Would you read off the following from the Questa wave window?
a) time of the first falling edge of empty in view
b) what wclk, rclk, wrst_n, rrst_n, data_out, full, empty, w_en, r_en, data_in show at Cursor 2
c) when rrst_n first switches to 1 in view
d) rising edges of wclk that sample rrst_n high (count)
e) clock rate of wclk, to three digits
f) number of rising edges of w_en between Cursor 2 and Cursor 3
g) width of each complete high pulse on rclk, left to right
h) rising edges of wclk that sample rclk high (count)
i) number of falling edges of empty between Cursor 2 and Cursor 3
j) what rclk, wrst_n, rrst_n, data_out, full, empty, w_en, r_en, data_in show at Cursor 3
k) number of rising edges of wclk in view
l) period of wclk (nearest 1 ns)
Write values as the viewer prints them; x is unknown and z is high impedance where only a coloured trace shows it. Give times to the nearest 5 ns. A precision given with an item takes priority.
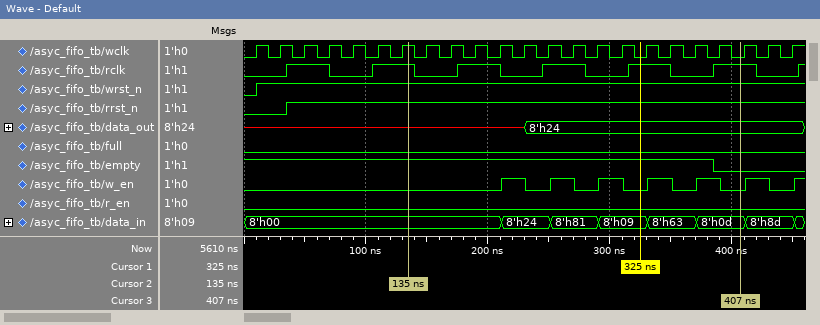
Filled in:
385 ns
wclk=1, rclk=1, wrst_n=1, rrst_n=1, data_out=x, full=0, empty=1, w_en=0, r_en=0, data_in=8'h00
35 ns
21
50.0 MHz
5
35 ns, 35 ns, 35 ns, 35 ns, 35 ns, 35 ns
12
1
rclk=1, wrst_n=1, rrst_n=1, data_out=8'h24, full=0, empty=0, w_en=0, r_en=0, data_in=8'h0d
23
20 ns
